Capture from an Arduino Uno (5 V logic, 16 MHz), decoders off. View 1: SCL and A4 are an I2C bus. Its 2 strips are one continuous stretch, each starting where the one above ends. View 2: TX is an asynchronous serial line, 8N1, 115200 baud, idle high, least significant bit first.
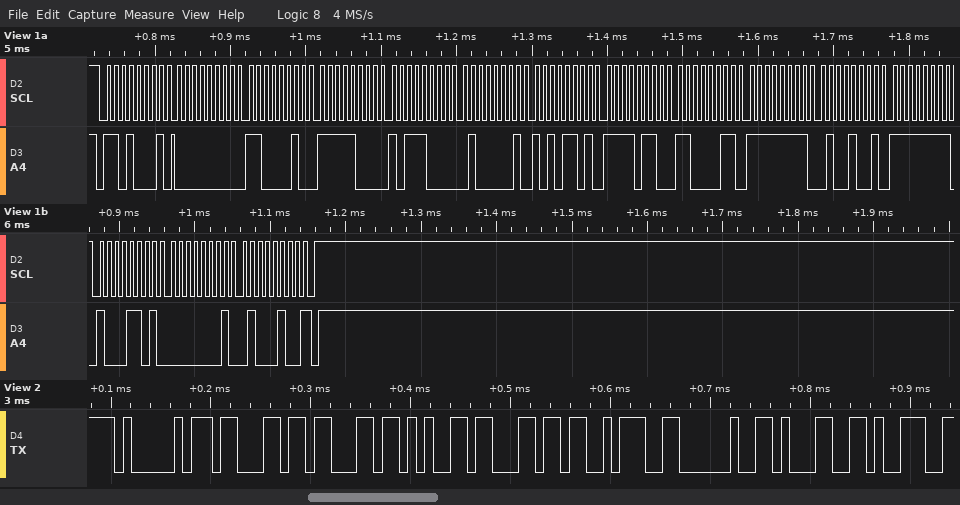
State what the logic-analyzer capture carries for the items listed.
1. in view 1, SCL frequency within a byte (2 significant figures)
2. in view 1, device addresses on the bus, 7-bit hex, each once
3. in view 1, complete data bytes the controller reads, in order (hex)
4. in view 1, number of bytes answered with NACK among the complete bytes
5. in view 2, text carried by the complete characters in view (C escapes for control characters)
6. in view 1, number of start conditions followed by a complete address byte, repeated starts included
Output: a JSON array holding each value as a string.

["100 kHz", "0x68", "00 C2 F8 B8 41 AD F6 C3 FF 49 FF 8D 01 44", "1", "\"Accel: 19\"", "1"]
